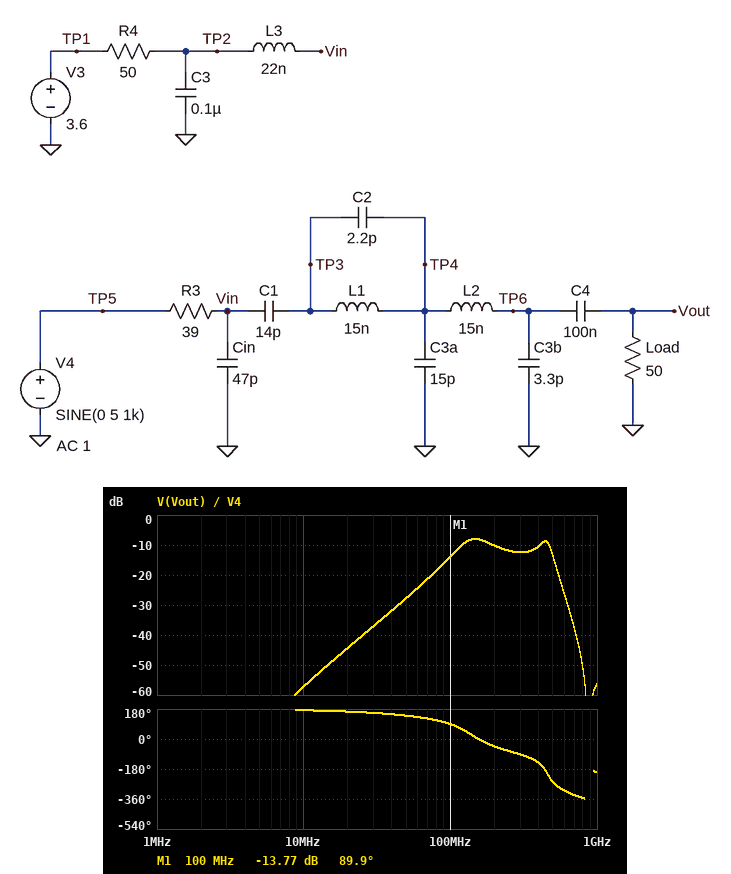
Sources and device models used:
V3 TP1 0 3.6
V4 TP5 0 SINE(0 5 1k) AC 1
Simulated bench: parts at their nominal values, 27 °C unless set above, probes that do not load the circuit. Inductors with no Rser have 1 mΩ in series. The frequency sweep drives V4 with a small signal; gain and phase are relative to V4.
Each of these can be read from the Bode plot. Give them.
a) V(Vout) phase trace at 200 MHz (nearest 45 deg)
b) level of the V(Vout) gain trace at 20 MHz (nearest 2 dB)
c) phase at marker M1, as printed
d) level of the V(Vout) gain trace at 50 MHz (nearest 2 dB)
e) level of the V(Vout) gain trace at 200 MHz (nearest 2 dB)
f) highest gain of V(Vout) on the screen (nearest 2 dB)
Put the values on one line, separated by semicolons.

-45 deg; -44 dB; 89.9 deg; -28 dB; -10 dB; -8 dB
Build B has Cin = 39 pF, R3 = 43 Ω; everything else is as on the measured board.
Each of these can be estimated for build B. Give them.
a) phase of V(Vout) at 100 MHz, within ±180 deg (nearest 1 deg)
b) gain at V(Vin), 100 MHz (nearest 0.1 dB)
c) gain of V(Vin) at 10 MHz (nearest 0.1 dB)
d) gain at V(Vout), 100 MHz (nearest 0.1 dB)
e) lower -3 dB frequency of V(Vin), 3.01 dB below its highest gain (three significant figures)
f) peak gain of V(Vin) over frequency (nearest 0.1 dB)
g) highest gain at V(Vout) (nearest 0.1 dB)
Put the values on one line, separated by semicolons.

96 deg; -6.3 dB; -30.9 dB; -15.1 dB; 112 MHz; -1.6 dB; -7.8 dB
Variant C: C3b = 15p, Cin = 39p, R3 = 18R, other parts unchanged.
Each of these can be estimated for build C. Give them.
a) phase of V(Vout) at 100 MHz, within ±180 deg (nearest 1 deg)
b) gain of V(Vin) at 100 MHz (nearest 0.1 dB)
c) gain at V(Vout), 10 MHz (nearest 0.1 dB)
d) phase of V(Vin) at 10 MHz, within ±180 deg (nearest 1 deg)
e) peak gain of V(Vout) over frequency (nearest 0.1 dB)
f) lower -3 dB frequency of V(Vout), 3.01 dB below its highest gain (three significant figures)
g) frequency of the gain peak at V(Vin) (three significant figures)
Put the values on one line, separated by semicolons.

67 deg; -2.0 dB; -50.5 dB; 86 deg; -2.6 dB; 251 MHz; 145 MHz
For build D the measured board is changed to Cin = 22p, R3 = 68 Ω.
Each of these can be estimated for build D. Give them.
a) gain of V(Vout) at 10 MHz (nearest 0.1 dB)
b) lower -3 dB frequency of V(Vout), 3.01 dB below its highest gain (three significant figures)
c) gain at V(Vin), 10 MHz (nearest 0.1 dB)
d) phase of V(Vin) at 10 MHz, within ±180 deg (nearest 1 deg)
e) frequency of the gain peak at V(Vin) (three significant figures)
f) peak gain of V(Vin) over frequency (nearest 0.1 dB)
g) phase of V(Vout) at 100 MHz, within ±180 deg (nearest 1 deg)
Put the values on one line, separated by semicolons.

-62.0 dB; 152 MHz; -34.9 dB; 89 deg; 183 MHz; -3.0 dB; 110 deg
